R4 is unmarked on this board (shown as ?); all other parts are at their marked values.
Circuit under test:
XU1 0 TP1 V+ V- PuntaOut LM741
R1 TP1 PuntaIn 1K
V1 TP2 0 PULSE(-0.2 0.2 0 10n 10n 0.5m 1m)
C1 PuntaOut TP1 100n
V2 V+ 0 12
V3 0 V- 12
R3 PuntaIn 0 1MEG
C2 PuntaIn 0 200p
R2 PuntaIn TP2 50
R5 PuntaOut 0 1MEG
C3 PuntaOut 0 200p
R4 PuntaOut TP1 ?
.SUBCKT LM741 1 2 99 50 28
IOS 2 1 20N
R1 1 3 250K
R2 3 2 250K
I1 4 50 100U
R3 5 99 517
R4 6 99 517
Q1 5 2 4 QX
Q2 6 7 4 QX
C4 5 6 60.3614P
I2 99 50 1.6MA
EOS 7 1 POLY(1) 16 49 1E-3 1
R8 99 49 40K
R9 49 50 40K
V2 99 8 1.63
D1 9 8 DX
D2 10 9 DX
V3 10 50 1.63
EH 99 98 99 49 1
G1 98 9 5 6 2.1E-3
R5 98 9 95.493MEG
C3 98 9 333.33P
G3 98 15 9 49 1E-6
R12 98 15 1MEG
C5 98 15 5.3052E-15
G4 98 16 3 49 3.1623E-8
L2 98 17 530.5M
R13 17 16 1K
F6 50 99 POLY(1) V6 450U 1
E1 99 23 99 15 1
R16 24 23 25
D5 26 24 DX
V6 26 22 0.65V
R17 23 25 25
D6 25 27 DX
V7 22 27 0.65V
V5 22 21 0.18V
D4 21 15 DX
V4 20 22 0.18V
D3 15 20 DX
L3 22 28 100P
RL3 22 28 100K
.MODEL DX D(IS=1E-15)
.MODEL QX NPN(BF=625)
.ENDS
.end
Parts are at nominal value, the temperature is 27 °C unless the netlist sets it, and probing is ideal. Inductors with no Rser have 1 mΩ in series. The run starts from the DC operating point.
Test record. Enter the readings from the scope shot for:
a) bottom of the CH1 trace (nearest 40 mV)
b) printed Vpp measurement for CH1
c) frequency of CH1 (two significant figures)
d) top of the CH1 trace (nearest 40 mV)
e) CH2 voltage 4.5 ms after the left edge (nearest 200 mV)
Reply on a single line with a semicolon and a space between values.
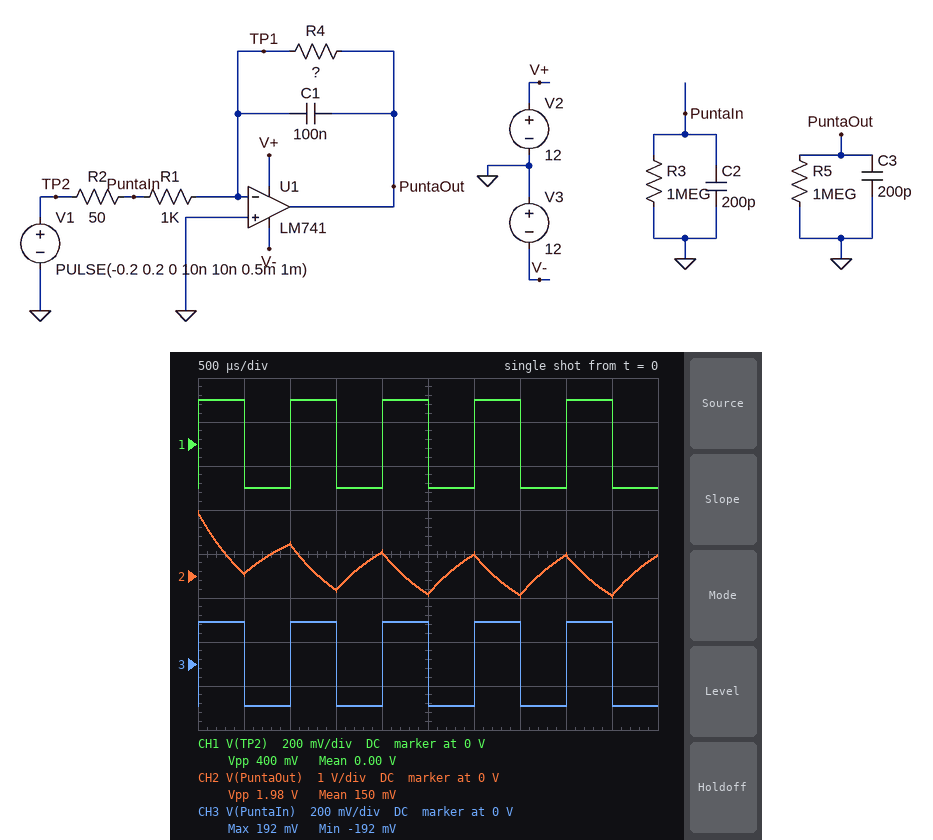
-200 mV; 400 mV; 1.0 kHz; 200 mV; -400 mV
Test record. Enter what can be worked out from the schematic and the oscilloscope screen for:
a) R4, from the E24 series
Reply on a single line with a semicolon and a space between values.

7.5 kΩ
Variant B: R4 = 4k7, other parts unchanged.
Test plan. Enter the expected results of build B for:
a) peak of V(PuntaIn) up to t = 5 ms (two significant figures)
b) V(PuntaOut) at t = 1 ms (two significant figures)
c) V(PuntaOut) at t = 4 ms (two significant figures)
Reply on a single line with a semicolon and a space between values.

190 mV; 500 mV; 440 mV
